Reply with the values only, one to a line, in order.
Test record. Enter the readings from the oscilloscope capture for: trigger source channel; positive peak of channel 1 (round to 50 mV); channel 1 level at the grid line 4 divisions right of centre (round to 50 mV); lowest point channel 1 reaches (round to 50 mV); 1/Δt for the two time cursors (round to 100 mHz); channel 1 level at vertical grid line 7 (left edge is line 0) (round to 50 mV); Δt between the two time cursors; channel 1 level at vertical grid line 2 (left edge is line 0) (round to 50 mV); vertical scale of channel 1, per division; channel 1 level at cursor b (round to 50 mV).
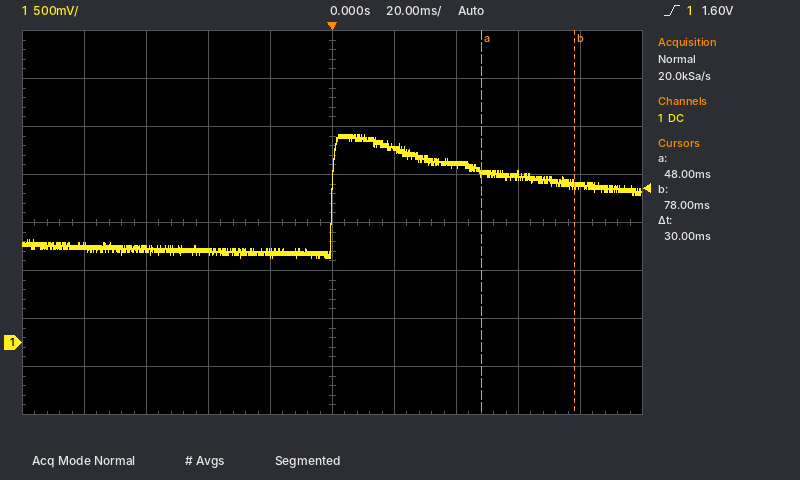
channel 1
2.15 V
1.65 V
900 mV
33.3 Hz
1.85 V
30 ms
1.00 V
500 mV
1.65 V
